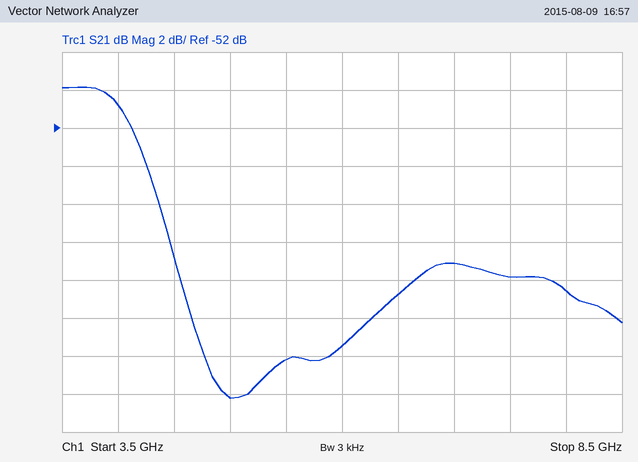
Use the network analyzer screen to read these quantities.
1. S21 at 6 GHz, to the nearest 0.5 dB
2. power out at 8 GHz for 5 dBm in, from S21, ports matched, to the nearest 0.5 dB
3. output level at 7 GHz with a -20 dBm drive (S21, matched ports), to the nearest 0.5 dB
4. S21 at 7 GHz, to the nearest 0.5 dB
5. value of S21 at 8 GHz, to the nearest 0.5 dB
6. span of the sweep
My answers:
-63.5 dB
-55.5 dBm
-79.0 dBm
-59.0 dB
-60.5 dB
5 GHz
